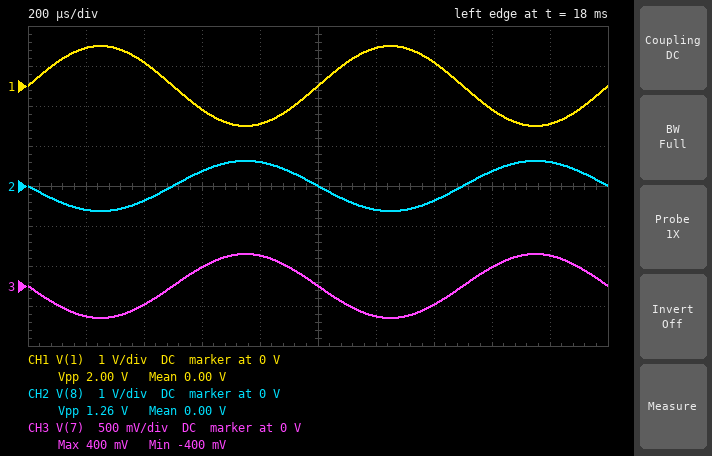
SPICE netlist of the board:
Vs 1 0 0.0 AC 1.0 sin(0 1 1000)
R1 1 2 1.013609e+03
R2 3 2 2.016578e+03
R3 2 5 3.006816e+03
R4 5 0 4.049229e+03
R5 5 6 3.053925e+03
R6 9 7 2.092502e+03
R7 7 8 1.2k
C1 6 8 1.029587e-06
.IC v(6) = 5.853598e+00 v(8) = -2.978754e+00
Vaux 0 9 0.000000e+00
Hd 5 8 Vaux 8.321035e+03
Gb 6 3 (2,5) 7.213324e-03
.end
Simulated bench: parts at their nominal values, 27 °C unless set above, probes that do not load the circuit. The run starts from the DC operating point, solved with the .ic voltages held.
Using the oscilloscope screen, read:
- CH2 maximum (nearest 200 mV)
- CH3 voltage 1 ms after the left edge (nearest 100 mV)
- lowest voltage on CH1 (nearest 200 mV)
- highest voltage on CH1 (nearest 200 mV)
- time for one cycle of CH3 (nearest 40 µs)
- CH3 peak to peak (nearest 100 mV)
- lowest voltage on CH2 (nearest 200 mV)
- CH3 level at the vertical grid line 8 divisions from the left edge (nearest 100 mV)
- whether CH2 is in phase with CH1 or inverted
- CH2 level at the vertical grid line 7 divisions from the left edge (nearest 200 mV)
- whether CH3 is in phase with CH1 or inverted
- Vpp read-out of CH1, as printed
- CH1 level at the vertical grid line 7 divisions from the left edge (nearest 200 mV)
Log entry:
600 mV
0 V
-1.0 V
1.0 V
1.00 ms
800 mV
-600 mV
200 mV
inverted
-400 mV
inverted
2.00 V
600 mV
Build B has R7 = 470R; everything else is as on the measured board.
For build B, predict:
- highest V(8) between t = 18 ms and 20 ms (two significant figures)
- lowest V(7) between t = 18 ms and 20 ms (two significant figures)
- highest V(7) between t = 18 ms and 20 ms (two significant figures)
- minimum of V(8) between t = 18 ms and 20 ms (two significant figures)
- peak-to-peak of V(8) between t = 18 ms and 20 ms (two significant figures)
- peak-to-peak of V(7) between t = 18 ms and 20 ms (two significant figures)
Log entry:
420 mV
-340 mV
340 mV
-420 mV
840 mV
680 mV
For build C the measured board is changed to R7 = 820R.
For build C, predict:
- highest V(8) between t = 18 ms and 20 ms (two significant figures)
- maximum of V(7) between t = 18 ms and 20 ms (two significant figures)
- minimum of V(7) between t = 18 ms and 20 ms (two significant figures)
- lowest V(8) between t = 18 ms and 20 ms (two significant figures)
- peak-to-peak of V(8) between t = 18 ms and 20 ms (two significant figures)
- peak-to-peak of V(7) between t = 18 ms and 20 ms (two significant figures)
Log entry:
510 mV
370 mV
-370 mV
-510 mV
1.0 V
730 mV
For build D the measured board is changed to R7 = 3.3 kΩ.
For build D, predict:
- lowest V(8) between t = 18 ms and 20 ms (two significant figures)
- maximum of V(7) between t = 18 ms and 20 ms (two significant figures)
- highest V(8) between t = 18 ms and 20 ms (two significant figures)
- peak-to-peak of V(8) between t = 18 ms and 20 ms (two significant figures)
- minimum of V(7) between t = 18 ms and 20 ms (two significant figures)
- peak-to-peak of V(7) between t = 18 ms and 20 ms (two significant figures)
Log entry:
-2.0 V
780 mV
2.0 V
4.0 V
-780 mV
1.6 V
